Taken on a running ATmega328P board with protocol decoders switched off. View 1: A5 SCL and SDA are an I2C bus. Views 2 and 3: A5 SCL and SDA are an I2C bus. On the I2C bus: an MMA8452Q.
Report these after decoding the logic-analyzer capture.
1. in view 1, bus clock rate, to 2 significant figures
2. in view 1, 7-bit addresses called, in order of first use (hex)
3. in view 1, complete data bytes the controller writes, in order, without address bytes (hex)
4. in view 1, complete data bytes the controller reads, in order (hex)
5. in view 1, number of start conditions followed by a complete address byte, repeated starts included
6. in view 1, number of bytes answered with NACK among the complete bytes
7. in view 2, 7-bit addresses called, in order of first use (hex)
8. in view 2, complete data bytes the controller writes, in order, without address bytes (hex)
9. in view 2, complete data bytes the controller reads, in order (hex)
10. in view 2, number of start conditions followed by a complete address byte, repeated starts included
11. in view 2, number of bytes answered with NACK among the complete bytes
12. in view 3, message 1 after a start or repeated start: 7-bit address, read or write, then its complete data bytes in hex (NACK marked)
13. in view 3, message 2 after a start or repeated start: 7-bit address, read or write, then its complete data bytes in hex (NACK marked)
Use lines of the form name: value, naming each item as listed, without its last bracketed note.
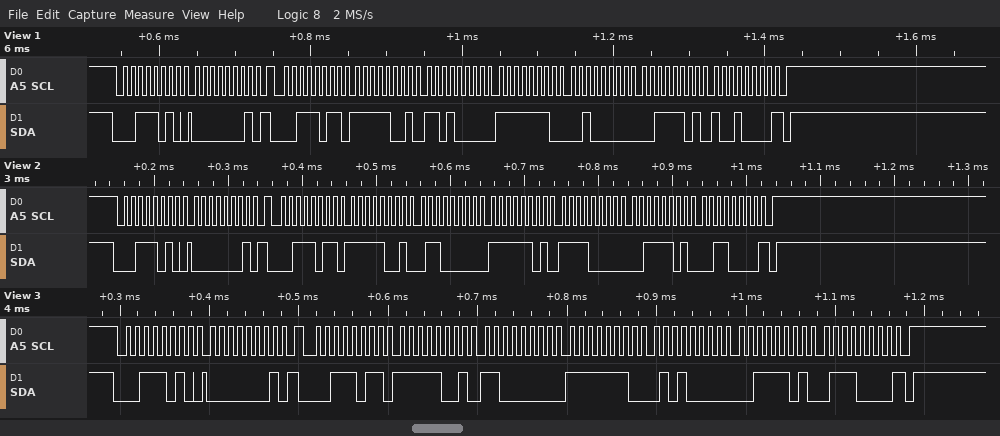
in view 1, bus clock rate, to 2 significant figures: 100 kHz
in view 1, 7-bit addresses called, in order of first use: 0x1D
in view 1, complete data bytes the controller writes, in order, without address bytes: 01
in view 1, complete data bytes the controller reads, in order: F9 D0 FE 20 3D 90
in view 1, number of start conditions followed by a complete address byte, repeated starts included: 2
in view 1, number of bytes answered with NACK among the complete bytes: 1
in view 2, 7-bit addresses called, in order of first use: 0x1D
in view 2, complete data bytes the controller writes, in order, without address bytes: 01
in view 2, complete data bytes the controller reads, in order: F9 60 FD F0 3D 30
in view 2, number of start conditions followed by a complete address byte, repeated starts included: 2
in view 2, number of bytes answered with NACK among the complete bytes: 1
in view 3, message 1 after a start or repeated start: 7-bit address, read or write, then its complete data bytes in hex: 0x1D write: 01
in view 3, message 2 after a start or repeated start: 7-bit address, read or write, then its complete data bytes in hex: 0x1D read: F9 C0 FE 50 3D 70 NACK
